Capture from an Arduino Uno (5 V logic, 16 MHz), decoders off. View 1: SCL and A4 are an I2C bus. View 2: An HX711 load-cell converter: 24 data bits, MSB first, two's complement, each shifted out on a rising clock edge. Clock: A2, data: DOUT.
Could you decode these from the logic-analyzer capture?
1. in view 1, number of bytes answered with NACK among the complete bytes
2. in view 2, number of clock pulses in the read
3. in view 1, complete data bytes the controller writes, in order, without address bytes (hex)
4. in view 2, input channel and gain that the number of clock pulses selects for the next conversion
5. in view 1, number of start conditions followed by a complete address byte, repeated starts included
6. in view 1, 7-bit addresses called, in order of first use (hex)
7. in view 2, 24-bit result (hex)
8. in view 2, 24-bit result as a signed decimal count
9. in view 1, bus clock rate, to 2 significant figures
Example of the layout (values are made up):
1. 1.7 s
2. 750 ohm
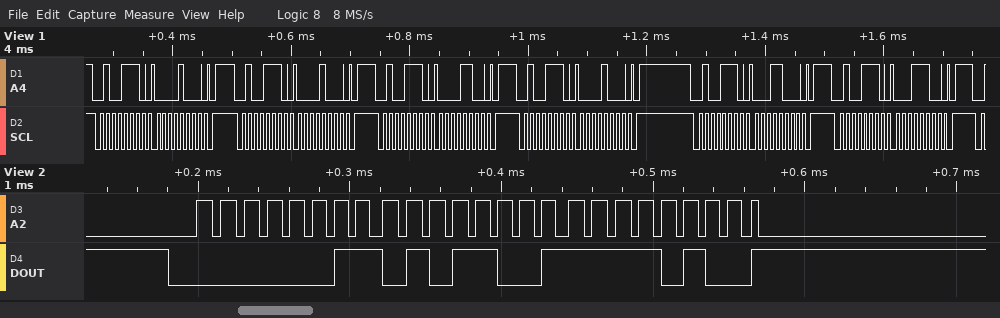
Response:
1. 0
2. 25
3. 08 08 0C 08 18 1C
4. channel A, gain 128
5. 6
6. 0x27
7. 0x0359F4
8. 219636
9. 100 kHz
